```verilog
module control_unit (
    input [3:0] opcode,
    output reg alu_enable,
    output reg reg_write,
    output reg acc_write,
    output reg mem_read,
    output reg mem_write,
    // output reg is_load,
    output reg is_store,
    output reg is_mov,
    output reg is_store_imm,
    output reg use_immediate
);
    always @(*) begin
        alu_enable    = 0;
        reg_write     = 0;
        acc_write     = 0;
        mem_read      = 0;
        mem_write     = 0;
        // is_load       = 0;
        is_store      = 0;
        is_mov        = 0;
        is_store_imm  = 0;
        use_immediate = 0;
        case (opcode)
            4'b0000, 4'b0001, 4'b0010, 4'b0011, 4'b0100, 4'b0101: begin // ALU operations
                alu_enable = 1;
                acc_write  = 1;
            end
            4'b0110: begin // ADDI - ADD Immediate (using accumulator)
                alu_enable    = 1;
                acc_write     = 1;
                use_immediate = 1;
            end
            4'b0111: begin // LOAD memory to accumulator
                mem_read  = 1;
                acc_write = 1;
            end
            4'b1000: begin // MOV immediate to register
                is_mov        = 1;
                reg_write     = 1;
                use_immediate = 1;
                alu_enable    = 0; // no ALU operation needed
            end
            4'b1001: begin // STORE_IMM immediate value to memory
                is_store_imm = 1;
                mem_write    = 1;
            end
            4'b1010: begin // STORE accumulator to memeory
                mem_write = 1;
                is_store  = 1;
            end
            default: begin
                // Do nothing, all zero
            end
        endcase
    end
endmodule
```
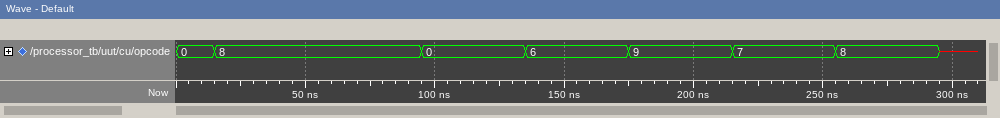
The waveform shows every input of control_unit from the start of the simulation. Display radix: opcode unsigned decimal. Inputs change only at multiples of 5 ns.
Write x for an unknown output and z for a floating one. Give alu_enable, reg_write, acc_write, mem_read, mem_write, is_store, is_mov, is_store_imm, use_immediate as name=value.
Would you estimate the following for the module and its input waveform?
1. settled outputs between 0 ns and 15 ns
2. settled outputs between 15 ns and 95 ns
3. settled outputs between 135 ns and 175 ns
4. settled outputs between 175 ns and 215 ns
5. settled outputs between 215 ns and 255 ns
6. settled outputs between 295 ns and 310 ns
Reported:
alu_enable=1, reg_write=0, acc_write=1, mem_read=0, mem_write=0, is_store=0, is_mov=0, is_store_imm=0, use_immediate=0
alu_enable=0, reg_write=1, acc_write=0, mem_read=0, mem_write=0, is_store=0, is_mov=1, is_store_imm=0, use_immediate=1
alu_enable=1, reg_write=0, acc_write=1, mem_read=0, mem_write=0, is_store=0, is_mov=0, is_store_imm=0, use_immediate=1
alu_enable=0, reg_write=0, acc_write=0, mem_read=0, mem_write=1, is_store=0, is_mov=0, is_store_imm=1, use_immediate=0
alu_enable=0, reg_write=0, acc_write=1, mem_read=1, mem_write=0, is_store=0, is_mov=0, is_store_imm=0, use_immediate=0
alu_enable=0, reg_write=0, acc_write=0, mem_read=0, mem_write=0, is_store=0, is_mov=0, is_store_imm=0, use_immediate=0
